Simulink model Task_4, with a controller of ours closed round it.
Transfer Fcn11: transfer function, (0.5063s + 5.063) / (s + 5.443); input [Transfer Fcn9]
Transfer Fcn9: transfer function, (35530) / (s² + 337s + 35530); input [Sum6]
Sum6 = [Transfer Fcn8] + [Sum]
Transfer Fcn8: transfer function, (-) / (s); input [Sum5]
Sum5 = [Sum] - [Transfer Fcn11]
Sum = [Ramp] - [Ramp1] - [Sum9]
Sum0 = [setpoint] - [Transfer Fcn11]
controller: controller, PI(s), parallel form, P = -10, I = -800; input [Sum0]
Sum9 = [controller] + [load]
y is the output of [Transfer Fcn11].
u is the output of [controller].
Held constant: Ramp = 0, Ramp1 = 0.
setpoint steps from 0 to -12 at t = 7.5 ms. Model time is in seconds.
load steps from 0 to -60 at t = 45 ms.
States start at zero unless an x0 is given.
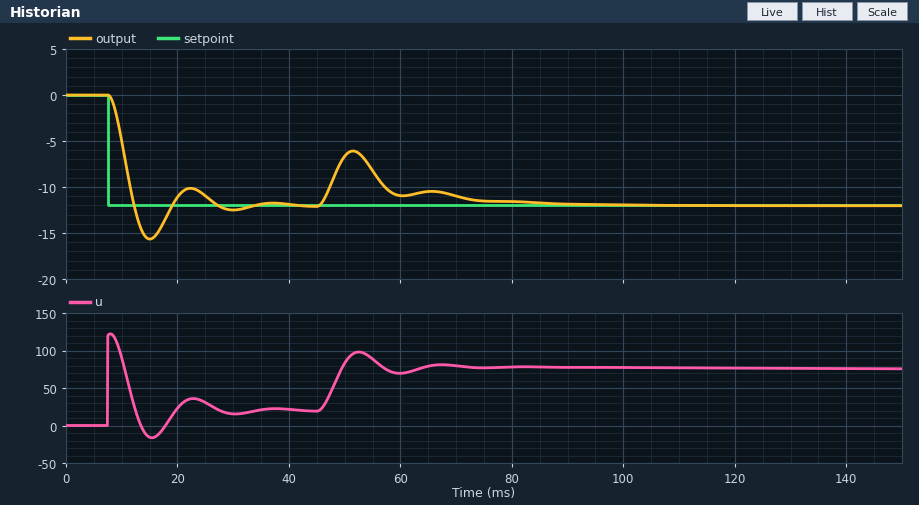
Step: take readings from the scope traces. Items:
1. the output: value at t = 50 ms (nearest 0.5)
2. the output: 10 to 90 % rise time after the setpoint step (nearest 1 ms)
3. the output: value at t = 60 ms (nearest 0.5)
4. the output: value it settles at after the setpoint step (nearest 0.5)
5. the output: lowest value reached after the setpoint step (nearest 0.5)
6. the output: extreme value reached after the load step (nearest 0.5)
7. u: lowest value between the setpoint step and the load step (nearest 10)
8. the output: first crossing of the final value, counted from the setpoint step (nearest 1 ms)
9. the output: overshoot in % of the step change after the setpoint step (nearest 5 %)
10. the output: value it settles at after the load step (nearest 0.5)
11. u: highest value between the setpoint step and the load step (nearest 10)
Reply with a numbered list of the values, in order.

1. -6.5
2. 3 ms
3. -11.0
4. -12.0
5. -15.5
6. -6.0
7. -20
8. 5 ms
9. 30 %
10. -12.0
11. 120
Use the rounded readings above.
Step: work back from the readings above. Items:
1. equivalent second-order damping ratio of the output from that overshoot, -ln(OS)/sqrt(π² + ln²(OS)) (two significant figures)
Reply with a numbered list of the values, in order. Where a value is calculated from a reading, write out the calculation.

1. ln(0.3) = -1.204; 1.204 / sqrt(9.870 + 1.450) = 0.36
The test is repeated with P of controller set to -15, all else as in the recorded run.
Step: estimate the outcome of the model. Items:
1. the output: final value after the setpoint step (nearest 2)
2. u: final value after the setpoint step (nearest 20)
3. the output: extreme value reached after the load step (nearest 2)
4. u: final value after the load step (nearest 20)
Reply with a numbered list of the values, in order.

1. -12
2. 20
3. -8
4. 80
